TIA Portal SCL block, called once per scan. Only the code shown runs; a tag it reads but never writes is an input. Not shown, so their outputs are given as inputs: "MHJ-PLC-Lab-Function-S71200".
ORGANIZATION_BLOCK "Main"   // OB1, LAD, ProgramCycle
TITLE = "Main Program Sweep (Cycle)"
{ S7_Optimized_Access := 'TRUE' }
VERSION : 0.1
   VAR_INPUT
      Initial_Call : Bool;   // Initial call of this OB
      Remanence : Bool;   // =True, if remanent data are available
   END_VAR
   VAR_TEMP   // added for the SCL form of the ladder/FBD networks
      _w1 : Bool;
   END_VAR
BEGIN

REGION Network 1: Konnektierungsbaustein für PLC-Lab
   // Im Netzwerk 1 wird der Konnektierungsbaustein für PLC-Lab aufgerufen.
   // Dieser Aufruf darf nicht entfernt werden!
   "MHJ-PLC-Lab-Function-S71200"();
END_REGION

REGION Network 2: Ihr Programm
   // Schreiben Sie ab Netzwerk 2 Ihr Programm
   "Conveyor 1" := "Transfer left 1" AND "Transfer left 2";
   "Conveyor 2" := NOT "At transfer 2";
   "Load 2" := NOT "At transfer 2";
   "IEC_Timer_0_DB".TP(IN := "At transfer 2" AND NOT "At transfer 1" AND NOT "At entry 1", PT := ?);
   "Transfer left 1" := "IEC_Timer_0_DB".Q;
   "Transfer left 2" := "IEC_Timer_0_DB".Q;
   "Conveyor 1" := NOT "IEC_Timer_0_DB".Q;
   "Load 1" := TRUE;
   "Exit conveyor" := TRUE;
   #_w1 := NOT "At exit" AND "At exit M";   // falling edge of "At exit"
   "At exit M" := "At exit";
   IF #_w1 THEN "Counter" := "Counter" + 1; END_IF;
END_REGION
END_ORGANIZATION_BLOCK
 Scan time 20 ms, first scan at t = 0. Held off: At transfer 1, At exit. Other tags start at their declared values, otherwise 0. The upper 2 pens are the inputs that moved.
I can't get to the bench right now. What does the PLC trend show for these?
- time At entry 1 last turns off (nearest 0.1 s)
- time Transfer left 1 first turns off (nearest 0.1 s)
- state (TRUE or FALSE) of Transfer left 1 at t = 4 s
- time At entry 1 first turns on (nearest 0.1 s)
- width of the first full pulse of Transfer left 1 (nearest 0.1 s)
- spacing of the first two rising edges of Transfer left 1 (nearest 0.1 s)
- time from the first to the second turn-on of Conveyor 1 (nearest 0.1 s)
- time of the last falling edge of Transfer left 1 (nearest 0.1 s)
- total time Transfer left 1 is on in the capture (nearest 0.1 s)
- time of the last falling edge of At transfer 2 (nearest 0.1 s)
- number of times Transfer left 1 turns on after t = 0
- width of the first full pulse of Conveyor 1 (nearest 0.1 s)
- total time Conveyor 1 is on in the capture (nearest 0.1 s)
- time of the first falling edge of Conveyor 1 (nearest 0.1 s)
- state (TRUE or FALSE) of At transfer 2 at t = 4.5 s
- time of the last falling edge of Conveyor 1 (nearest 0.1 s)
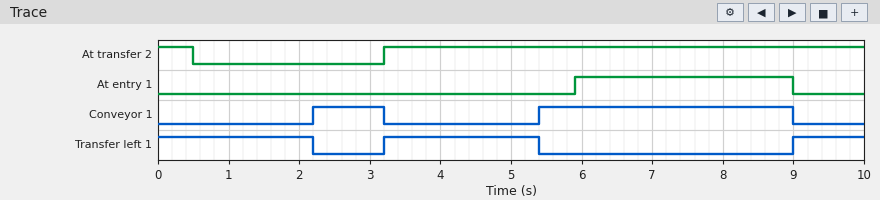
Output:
9.0 s
2.2 s
TRUE
5.9 s
2.2 s
5.8 s
3.2 s
5.4 s
5.4 s
0.5 s
2
1.0 s
4.6 s
3.2 s
TRUE
9.0 s
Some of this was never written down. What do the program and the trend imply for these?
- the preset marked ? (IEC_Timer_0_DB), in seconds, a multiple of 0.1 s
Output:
2.2 s
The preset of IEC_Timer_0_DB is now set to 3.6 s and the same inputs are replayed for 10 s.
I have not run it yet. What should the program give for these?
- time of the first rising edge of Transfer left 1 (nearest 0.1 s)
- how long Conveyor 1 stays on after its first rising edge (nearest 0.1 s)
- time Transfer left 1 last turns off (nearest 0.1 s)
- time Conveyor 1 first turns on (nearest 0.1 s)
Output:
9.0 s
5.4 s
3.6 s
3.6 s
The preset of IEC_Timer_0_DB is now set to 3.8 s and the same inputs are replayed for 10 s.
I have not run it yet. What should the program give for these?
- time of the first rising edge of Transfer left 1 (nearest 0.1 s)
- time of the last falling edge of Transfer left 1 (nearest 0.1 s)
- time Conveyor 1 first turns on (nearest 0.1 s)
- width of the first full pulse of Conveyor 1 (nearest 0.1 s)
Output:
9.0 s
3.8 s
3.8 s
5.2 s
